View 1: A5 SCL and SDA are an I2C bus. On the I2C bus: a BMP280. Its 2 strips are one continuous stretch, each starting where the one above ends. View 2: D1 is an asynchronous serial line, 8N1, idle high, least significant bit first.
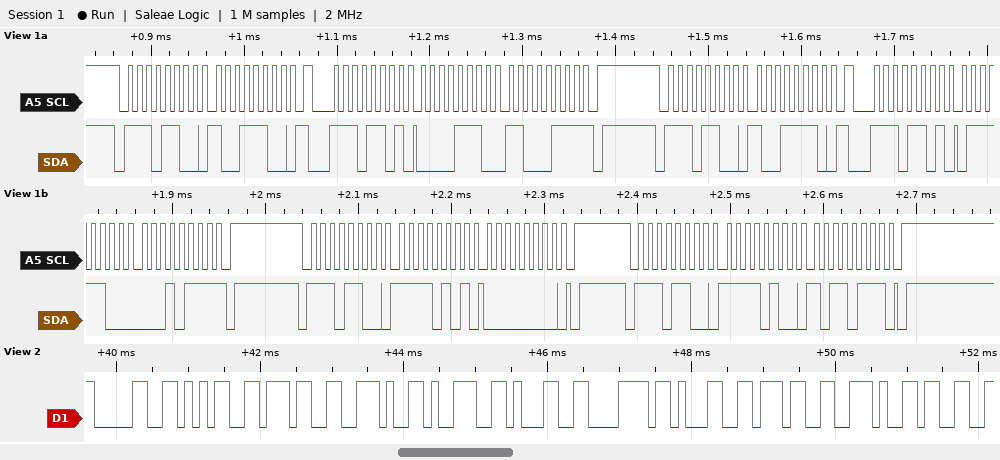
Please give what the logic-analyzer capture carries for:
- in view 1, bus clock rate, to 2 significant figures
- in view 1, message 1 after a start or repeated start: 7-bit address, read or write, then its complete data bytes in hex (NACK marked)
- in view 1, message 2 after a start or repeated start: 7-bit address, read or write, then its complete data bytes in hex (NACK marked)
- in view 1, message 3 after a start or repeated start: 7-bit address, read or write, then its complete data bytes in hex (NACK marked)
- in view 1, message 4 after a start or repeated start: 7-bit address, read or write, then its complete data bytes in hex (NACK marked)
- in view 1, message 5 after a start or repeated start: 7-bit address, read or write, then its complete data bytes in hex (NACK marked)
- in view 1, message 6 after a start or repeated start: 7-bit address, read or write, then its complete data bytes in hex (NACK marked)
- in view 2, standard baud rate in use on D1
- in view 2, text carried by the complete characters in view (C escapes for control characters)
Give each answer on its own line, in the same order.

100 kHz
0x76 write: 9C
0x76 read: 0E C7 NACK
0x76 write: 9E
0x76 read: 7C 17 NACK
0x76 write: F5 00
0x76 write: F4 B7
9600 baud
"057.91x17.3"
